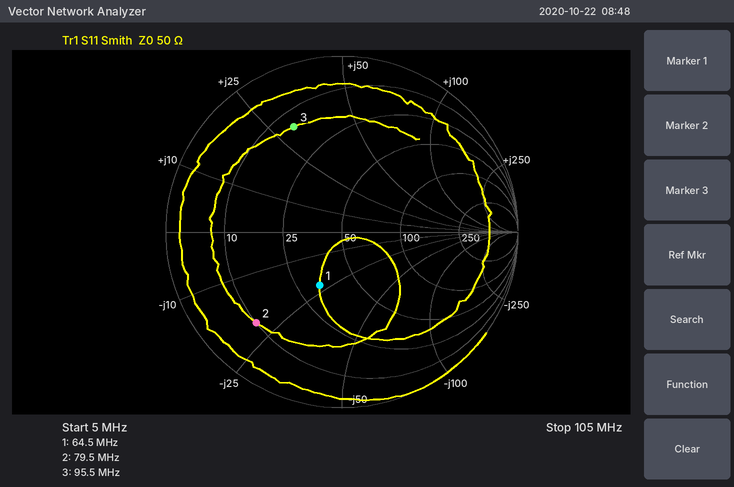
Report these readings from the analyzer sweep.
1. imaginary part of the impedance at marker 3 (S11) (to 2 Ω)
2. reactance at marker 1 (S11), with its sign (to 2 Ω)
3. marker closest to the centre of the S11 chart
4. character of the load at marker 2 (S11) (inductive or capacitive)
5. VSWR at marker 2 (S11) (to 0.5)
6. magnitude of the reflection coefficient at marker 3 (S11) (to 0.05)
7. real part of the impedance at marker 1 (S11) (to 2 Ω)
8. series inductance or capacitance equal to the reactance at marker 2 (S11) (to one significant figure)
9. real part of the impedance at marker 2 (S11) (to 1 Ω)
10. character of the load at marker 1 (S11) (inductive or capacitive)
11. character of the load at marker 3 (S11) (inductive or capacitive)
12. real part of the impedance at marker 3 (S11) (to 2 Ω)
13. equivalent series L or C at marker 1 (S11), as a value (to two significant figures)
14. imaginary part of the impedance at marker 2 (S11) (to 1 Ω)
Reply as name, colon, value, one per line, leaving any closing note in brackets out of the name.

imaginary part of the impedance at marker 3 (S11): +30 Ω
reactance at marker 1 (S11), with its sign: -22 Ω
marker closest to the centre of the S11 chart: marker 1
character of the load at marker 2 (S11): capacitive
VSWR at marker 2 (S11): 6.0
magnitude of the reflection coefficient at marker 3 (S11): 0.65
real part of the impedance at marker 1 (S11): 32 Ω
series inductance or capacitance equal to the reactance at marker 2 (S11): 100 pF
real part of the impedance at marker 2 (S11): 10 Ω
character of the load at marker 1 (S11): capacitive
character of the load at marker 3 (S11): inductive
real part of the impedance at marker 3 (S11): 14 Ω
equivalent series L or C at marker 1 (S11), as a value: 110 pF
imaginary part of the impedance at marker 2 (S11): -21 Ω
